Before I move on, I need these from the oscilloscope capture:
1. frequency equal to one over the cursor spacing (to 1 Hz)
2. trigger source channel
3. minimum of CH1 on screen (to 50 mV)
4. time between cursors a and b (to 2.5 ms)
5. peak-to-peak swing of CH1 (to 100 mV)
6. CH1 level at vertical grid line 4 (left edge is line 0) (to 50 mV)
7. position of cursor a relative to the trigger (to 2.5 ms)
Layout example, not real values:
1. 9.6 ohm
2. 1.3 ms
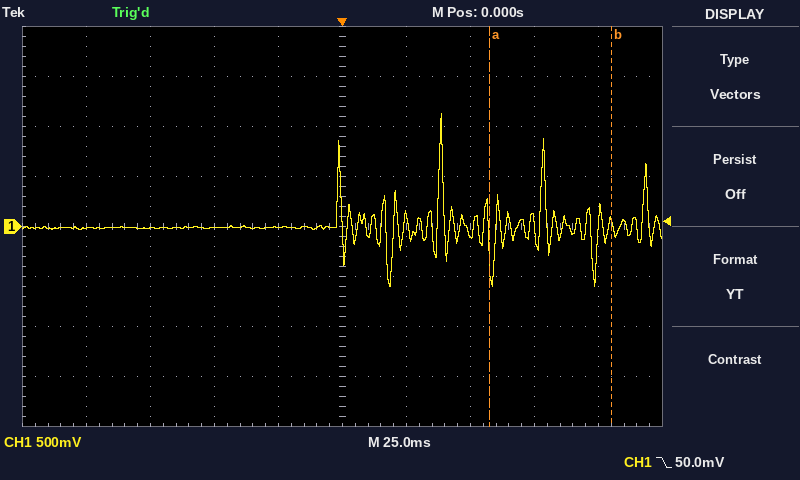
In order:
1. 21 Hz
2. CH1
3. -600 mV
4. 47.5 ms
5. 1.70 V
6. 0 mV
7. +57.5 ms
